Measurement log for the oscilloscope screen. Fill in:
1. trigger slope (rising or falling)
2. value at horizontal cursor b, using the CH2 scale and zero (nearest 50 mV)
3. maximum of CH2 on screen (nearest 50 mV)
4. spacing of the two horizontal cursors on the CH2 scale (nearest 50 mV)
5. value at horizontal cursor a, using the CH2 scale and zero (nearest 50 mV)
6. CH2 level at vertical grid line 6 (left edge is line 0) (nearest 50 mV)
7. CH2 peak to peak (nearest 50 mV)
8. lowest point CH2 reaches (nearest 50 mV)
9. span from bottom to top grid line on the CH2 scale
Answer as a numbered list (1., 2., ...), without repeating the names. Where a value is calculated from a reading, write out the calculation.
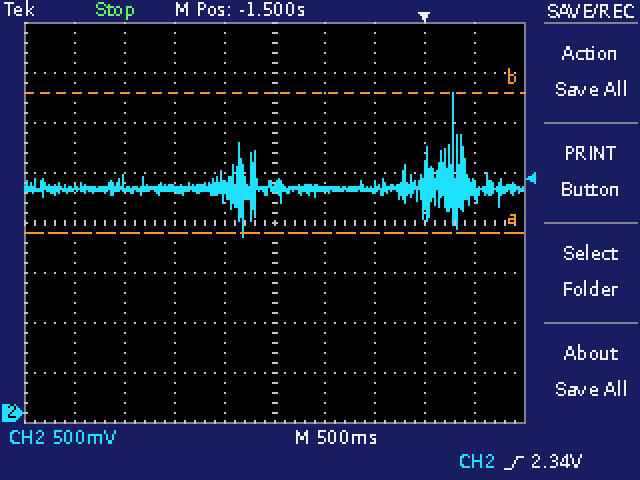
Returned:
1. rising
2. 3.20 V
3. 3.20 V
4. 1.40 V
5. 1.80 V
6. 2.25 V
7. 3.20 V − (1.75 V) = 1.45 V
8. 1.75 V
9. 4 V
